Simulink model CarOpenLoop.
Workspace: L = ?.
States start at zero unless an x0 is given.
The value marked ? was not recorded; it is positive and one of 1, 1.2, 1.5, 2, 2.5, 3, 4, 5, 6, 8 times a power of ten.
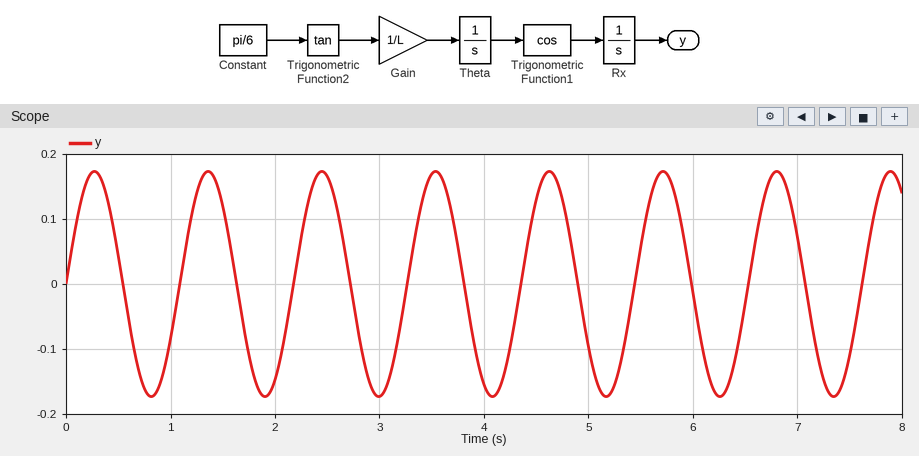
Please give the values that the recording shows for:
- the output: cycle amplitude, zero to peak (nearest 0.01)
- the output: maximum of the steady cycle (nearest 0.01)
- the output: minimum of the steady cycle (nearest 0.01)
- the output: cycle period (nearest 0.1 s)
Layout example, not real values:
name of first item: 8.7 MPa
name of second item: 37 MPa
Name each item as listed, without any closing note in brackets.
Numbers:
the output: cycle amplitude, zero to peak: 0.17
the output: maximum of the steady cycle: 0.17
the output: minimum of the steady cycle: -0.17
the output: cycle period: 1.1 s
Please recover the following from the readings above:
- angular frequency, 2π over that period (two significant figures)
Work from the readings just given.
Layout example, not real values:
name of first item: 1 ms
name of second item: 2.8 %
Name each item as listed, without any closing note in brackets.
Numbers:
angular frequency, 2π over that period: 5.7 rad/s
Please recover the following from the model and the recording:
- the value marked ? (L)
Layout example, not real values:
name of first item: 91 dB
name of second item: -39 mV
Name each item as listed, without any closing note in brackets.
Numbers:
the value marked ?: 0.1
